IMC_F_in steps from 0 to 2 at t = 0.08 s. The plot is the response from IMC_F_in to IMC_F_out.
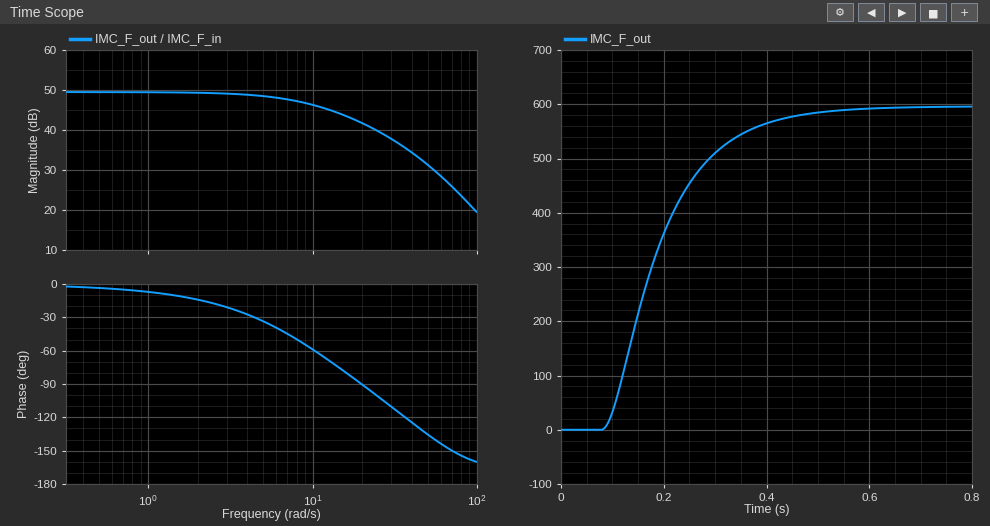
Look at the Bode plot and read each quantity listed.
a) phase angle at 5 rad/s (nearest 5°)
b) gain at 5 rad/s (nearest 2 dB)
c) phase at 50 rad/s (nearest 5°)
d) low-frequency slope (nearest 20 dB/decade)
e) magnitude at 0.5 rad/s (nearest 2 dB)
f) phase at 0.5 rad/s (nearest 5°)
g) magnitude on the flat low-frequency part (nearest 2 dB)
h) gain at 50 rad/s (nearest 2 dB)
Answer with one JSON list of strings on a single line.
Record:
["-35°", "48 dB", "-135°", "0 dB/decade", "50 dB", "-5°", "50 dB", "32 dB"]
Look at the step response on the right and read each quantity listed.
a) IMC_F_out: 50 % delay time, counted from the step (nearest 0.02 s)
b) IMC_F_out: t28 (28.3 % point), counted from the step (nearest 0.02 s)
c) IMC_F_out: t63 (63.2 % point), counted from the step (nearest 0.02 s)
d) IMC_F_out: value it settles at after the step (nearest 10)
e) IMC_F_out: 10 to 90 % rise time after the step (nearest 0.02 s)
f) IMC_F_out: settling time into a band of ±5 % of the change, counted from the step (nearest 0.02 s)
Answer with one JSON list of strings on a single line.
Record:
["0.10 s", "0.06 s", "0.12 s", "600", "0.22 s", "0.32 s"]
